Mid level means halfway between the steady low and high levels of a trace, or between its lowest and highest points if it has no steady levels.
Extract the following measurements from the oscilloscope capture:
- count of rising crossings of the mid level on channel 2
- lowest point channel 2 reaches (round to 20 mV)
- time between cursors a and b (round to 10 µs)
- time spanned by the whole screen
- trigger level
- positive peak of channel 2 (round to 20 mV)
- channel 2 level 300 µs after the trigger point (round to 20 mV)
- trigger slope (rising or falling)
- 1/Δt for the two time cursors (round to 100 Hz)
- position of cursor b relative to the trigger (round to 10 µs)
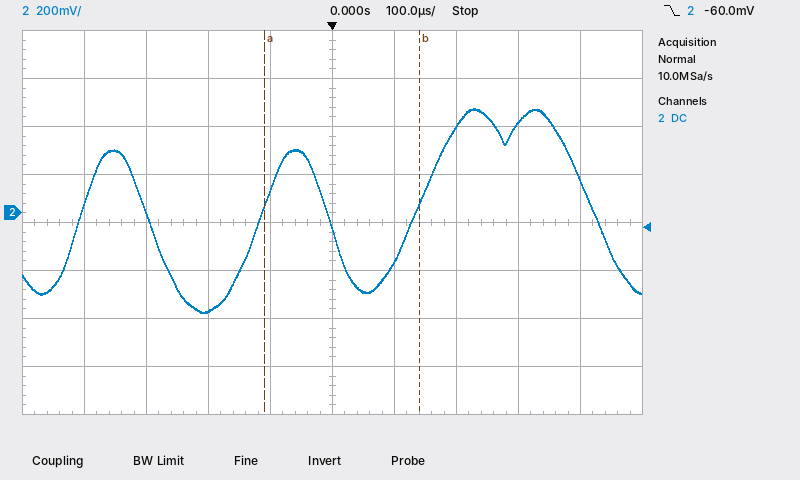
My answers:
3
-420 mV
250 µs
1 ms
-60.0 mV
440 mV
380 mV
falling
4.0 kHz
+140 µs
